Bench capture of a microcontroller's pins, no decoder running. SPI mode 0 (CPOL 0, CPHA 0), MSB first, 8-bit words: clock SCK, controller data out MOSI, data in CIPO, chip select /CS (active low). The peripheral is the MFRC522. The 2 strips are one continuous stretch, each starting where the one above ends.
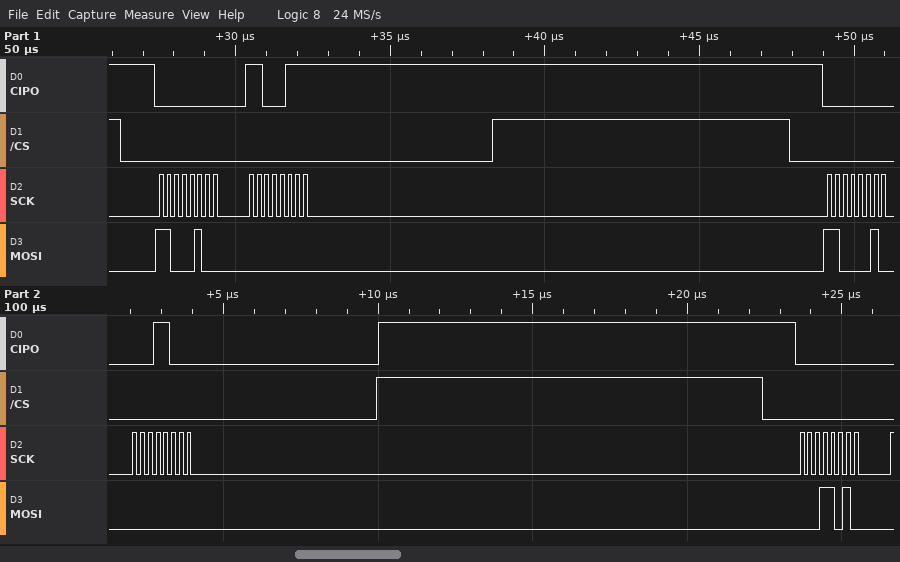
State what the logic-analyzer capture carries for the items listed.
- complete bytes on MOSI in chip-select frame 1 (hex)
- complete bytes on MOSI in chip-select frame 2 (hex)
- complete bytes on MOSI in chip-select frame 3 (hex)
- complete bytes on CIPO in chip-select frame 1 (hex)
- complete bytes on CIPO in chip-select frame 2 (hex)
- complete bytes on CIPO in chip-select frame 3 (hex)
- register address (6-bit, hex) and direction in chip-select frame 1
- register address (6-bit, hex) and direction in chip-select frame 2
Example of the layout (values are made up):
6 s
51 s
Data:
C4 00
C2 00
1A
00 C7
00 18
00
0x22 read
0x21 read
